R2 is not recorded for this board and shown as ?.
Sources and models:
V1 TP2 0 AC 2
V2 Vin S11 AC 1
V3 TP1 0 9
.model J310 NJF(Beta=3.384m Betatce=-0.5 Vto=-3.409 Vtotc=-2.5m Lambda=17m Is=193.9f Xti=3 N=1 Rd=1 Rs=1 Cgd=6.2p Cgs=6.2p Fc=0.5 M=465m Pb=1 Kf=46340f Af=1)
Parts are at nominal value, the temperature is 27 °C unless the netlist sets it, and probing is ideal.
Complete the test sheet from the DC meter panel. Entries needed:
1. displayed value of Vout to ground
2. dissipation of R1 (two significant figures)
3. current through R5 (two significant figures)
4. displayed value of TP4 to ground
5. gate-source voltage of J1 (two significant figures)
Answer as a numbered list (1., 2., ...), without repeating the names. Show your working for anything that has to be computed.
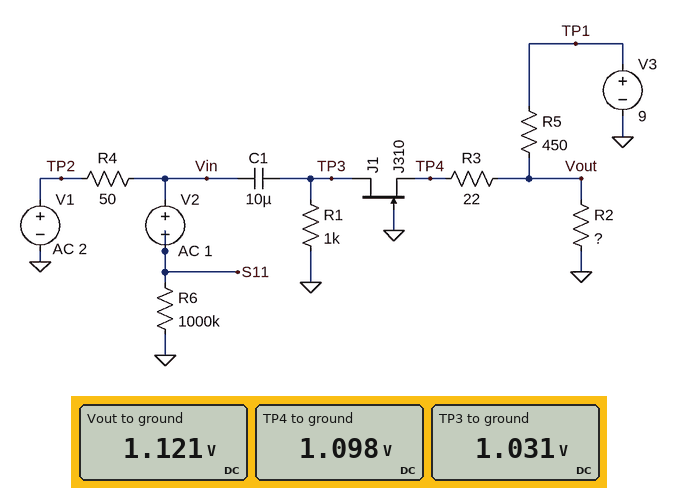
1. 1.121 V
2. (1.031 V)^2 / 1 kΩ = 1.1 mW
3. (9 V - 1.121 V) / 450 Ω = 18 mA
4. 1.098 V
5. 0 V - 1.098 V = -1.1 V
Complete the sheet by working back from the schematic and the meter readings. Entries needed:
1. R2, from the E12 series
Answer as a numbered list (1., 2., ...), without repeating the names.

1. 68 Ω
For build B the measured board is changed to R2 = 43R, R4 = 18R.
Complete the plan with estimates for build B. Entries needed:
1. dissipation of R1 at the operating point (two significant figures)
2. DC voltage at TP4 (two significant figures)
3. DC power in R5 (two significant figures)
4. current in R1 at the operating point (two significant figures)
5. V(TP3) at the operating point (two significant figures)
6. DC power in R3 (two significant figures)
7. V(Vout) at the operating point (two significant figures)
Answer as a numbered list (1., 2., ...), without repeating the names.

1. 490 µW
2. 740 mV
3. 150 mW
4. 700 µA
5. 700 mV
6. 11 µW
7. 760 mV
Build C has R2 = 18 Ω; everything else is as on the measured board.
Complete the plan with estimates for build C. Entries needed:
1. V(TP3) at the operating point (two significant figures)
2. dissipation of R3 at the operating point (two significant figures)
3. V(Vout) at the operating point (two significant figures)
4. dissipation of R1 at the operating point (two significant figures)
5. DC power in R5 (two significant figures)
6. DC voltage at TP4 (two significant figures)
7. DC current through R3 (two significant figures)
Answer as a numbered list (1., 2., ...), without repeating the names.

1. 320 mV
2. 2.2 µW
3. 340 mV
4. 100 µW
5. 170 mW
6. 330 mV
7. 320 µA
